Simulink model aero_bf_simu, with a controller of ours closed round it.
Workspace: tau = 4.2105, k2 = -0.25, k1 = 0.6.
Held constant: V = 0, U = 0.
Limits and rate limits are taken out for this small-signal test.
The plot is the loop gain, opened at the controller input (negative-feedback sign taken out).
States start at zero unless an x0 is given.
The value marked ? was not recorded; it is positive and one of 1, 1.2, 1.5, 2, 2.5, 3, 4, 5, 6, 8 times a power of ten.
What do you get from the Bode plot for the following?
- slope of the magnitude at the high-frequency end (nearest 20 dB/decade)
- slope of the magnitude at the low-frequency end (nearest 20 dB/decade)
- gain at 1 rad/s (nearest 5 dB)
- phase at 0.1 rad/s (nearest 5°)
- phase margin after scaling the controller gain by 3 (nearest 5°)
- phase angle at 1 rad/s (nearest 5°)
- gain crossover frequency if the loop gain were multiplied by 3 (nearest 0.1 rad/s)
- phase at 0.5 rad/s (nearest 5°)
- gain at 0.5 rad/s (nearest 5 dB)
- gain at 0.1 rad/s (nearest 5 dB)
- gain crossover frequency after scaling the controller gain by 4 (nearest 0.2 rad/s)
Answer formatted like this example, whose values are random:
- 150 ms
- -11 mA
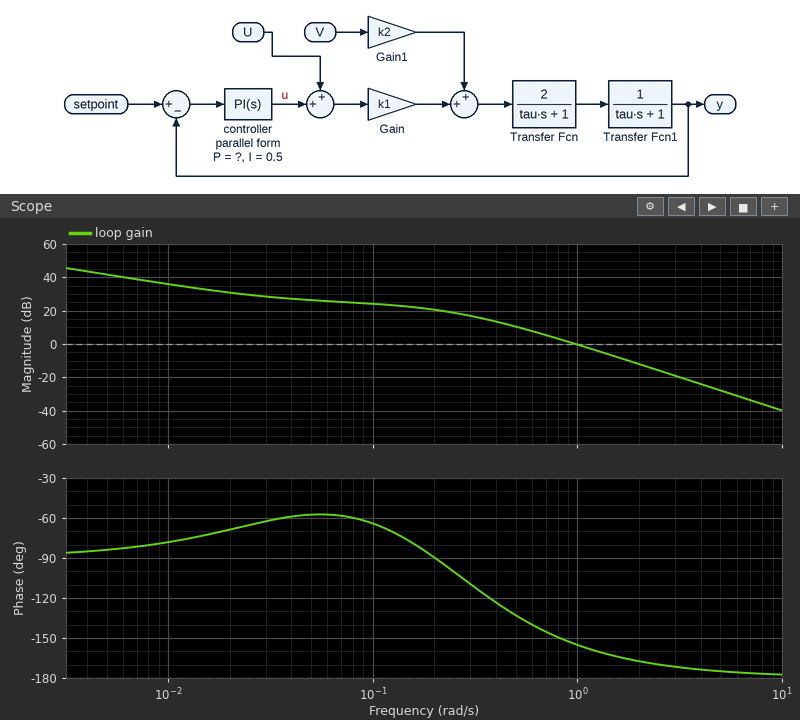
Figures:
- -40 dB/decade
- -20 dB/decade
- 0 dB
- -65°
- 15°
- -155°
- 1.7 rad/s
- -135°
- 10 dB
- 25 dB
- 2.0 rad/s
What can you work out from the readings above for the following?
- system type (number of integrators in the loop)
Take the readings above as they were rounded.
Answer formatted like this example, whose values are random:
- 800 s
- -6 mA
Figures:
- 1
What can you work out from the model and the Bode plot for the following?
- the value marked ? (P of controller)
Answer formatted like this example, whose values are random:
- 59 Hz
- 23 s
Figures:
- 15
